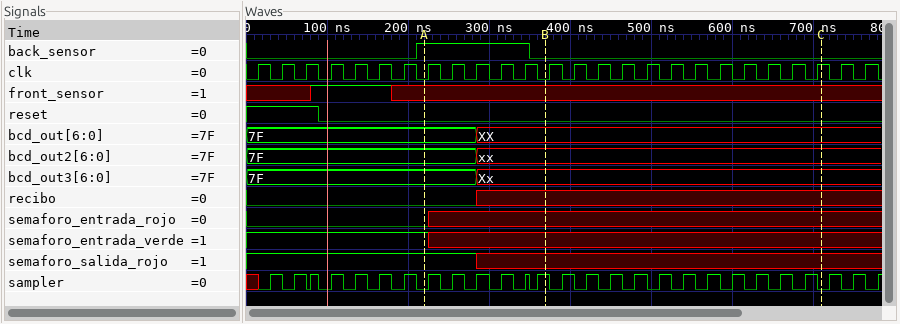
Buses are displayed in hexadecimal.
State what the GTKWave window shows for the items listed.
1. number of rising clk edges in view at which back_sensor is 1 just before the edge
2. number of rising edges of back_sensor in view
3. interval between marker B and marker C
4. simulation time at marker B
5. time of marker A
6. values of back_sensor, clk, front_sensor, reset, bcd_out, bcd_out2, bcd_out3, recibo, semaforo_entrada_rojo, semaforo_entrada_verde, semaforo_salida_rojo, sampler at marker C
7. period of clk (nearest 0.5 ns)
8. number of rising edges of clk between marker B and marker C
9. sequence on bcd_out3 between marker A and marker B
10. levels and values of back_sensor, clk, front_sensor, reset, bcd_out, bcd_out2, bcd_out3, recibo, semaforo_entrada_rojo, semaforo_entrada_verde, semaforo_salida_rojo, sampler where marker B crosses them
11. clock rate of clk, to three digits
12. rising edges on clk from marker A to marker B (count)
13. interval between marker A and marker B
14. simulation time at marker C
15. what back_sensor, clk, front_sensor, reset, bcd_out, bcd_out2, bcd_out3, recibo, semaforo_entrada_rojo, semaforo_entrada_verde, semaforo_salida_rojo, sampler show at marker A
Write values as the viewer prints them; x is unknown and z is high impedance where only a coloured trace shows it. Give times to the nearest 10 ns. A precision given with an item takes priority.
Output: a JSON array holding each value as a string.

["5", "1", "340 ns", "370 ns", "220 ns", "back_sensor=0, clk=1, front_sensor=x, reset=0, bcd_out=XX, bcd_out2=xx, bcd_out3=Xx, recibo=x, semaforo_entrada_rojo=x, semaforo_entrada_verde=x, semaforo_salida_rojo=x, sampler=0", "30 ns", "12", "7F, Xx", "back_sensor=0, clk=0, front_sensor=x, reset=0, bcd_out=XX, bcd_out2=xx, bcd_out3=Xx, recibo=x, semaforo_entrada_rojo=x, semaforo_entrada_verde=x, semaforo_salida_rojo=x, sampler=1", "33.3 MHz", "5", "150 ns", "710 ns", "back_sensor=1, clk=0, front_sensor=x, reset=0, bcd_out=7F, bcd_out2=7F, bcd_out3=7F, recibo=0, semaforo_entrada_rojo=0, semaforo_entrada_verde=1, semaforo_salida_rojo=1, sampler=0"]
